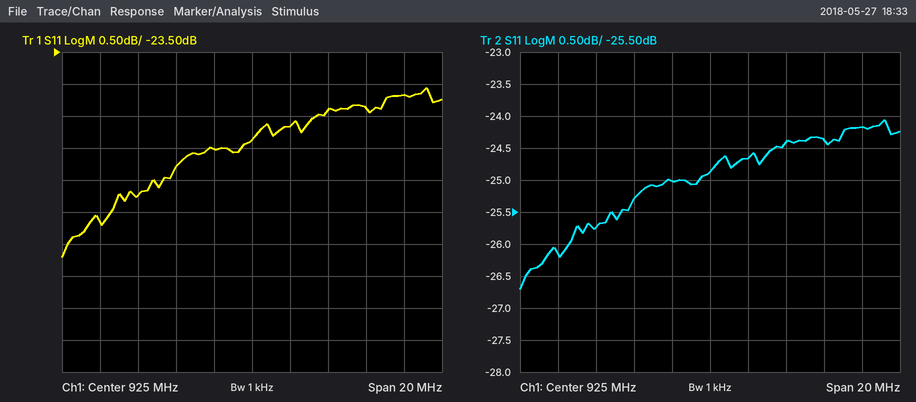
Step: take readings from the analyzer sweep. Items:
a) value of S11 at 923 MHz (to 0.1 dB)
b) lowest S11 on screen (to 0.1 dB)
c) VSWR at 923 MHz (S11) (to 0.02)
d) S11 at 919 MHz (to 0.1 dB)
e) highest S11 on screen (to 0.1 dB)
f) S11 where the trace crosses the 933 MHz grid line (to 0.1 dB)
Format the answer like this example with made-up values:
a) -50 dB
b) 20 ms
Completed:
a) -25.0 dB
b) -26.7 dB
c) 1.12
d) -25.7 dB
e) -24.1 dB
f) -24.2 dB
